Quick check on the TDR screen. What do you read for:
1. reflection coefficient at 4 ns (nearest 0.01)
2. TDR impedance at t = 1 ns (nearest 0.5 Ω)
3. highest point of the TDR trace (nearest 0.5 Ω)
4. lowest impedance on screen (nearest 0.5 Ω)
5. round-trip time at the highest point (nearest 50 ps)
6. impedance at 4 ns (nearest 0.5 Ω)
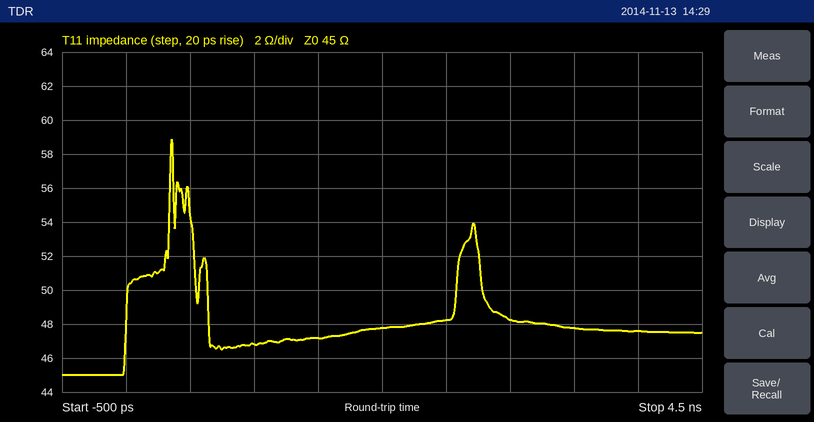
+0.03
47.0 Ω
59.0 Ω
45.0 Ω
350 ps
47.5 Ω
